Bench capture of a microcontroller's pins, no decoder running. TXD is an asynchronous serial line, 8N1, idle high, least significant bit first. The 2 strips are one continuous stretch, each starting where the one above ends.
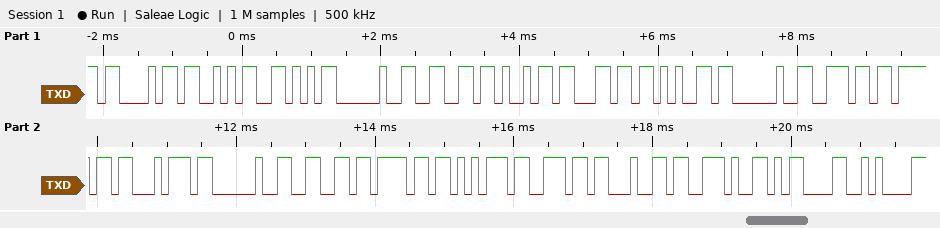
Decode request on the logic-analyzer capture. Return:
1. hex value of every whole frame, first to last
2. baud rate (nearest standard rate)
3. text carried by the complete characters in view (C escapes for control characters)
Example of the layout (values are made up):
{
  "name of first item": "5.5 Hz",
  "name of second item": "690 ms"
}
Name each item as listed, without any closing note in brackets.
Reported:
{
  "hex value of every whole frame, first to last": "0x43 0x53 0x56 0x20 0x66 0x69 0x6C 0x65 0x20 0x6E 0x6F 0x74 0x20 0x66 0x6F 0x75 0x6E 0x64 0x2E 0x0D 0x0A",
  "baud rate": "9600 baud",
  "text carried by the complete characters in view": "\"CSV file not found.\\r\\n\""
}
